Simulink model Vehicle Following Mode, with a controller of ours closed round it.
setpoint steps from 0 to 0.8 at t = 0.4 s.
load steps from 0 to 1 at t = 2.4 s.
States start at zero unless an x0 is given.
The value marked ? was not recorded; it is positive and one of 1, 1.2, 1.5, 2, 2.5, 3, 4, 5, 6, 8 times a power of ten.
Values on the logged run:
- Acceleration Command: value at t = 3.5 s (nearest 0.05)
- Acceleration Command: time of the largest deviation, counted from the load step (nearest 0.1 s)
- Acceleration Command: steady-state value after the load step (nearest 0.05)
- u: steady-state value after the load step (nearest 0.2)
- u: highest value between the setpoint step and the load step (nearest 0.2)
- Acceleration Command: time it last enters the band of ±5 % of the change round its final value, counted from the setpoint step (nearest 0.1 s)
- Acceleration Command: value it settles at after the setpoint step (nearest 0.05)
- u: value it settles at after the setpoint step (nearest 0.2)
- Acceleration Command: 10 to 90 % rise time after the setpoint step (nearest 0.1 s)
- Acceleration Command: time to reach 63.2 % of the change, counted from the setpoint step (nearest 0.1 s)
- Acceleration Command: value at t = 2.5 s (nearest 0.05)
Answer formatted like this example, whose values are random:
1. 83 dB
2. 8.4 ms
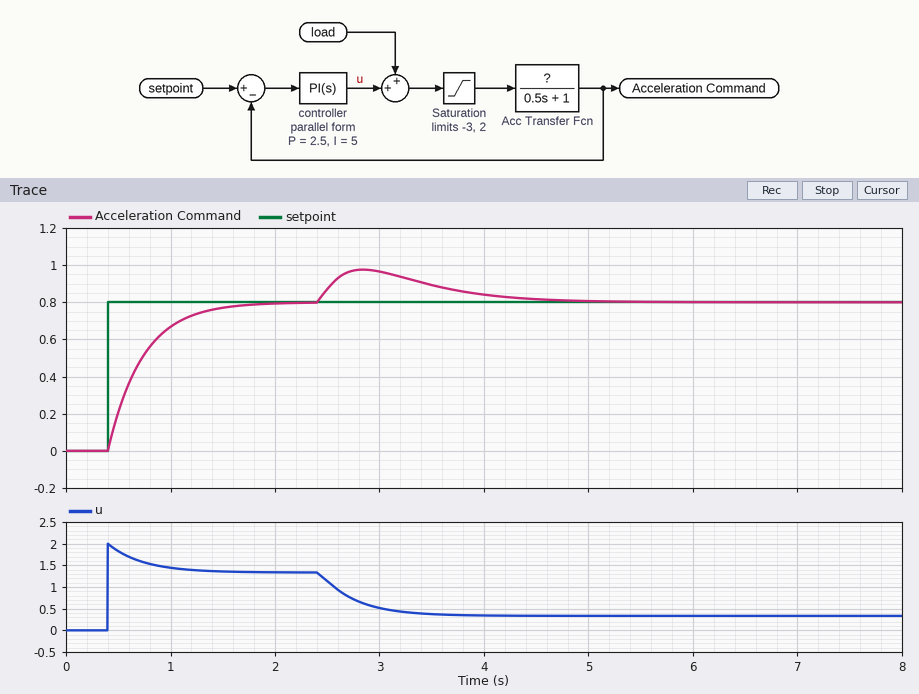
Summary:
1. 0.90
2. 0.4 s
3. 0.80
4. 0.4
5. 2.0
6. 1.0 s
7. 0.80
8. 1.4
9. 0.7 s
10. 0.3 s
11. 0.85
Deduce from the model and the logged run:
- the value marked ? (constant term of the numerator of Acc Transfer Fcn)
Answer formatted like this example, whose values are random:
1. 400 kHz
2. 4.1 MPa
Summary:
1. 0.6
